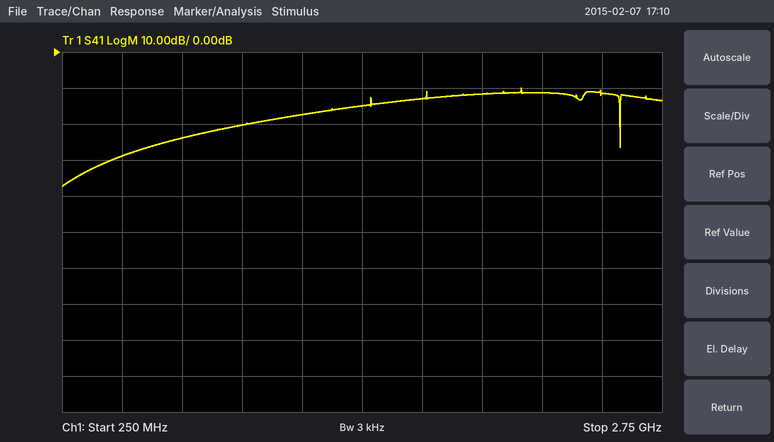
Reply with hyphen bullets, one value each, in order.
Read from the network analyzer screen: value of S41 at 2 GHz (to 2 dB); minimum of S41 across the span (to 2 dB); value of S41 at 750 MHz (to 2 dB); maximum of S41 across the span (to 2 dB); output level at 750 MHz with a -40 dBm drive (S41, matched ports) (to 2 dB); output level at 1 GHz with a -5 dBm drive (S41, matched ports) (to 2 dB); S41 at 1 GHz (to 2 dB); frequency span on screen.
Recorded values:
- -12 dB
- -38 dB
- -24 dB
- -10 dB
- -64 dBm
- -26 dBm
- -20 dB
- 2.5 GHz
